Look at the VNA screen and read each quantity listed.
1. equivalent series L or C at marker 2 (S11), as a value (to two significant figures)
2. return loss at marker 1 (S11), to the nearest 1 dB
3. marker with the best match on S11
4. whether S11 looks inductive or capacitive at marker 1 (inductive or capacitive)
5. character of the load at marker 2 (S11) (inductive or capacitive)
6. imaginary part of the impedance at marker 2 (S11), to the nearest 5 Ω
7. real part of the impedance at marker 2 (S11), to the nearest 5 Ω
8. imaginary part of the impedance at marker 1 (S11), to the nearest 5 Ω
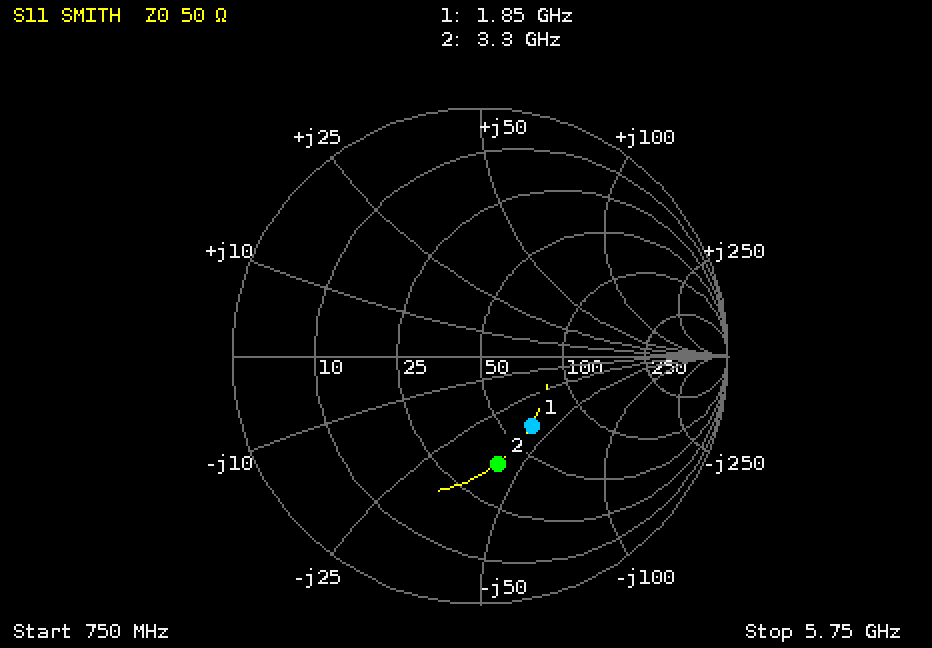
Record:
1.2 pF
9 dB
marker 1
capacitive
capacitive
-40 Ω
40 Ω
-40 Ω
